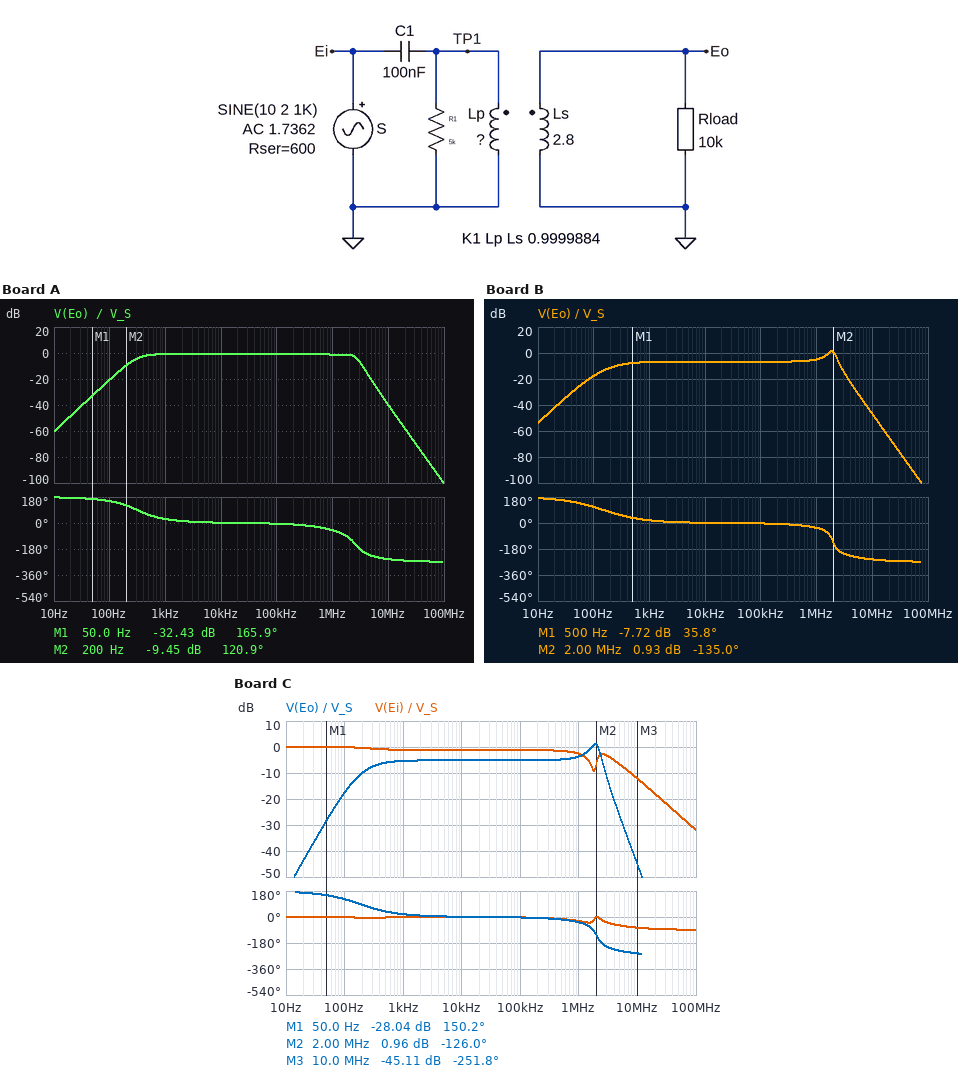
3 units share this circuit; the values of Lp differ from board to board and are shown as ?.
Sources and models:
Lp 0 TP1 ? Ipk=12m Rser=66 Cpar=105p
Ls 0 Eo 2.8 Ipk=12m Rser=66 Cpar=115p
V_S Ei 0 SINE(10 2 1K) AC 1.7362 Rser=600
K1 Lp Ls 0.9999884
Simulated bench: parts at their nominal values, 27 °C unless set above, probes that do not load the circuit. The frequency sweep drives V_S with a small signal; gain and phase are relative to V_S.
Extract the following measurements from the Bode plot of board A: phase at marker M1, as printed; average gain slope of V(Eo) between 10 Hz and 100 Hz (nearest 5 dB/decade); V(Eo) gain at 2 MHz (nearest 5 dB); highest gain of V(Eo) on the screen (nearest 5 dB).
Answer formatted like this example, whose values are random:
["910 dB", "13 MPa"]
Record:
["165.9 deg", "40 dB/decade", "0 dB", "0 dB"]
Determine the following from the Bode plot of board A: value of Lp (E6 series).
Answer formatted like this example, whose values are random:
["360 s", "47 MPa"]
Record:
["2.2 H"]
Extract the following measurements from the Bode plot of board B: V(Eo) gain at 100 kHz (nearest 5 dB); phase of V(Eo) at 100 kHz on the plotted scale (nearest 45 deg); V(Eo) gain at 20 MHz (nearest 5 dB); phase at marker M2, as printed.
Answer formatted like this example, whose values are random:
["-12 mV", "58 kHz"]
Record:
["-5 dB", "0 deg", "-65 dB", "-135.0 deg"]
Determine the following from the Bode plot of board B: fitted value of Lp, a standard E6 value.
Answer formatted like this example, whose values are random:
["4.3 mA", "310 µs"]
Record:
["10 H"]
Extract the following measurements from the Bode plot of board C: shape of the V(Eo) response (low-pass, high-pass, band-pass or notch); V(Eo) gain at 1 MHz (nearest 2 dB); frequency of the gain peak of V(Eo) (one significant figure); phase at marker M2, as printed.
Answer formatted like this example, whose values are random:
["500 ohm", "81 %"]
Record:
["band-pass", "-4 dB", "2 MHz", "-126.0 deg"]
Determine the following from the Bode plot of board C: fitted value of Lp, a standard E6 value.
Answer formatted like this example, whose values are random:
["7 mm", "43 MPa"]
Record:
["6.8 H"]
